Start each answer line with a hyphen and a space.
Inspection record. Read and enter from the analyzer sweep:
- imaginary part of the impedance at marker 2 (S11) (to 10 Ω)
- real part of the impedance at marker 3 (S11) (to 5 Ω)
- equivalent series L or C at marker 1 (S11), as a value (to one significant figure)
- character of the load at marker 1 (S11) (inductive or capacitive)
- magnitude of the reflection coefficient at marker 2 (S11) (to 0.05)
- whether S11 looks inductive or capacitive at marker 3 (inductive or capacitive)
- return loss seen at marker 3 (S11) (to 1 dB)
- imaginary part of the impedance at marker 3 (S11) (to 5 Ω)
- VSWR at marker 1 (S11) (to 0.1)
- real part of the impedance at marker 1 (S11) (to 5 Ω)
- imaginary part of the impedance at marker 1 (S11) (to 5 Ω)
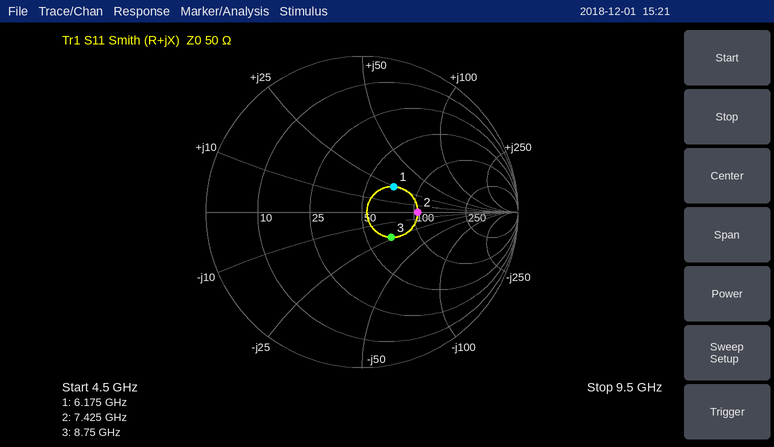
- 0 Ω
- 70 Ω
- 600 pH
- inductive
- 0.35
- capacitive
- 12 dB
- -25 Ω
- 1.7
- 70 Ω
- +25 Ω
